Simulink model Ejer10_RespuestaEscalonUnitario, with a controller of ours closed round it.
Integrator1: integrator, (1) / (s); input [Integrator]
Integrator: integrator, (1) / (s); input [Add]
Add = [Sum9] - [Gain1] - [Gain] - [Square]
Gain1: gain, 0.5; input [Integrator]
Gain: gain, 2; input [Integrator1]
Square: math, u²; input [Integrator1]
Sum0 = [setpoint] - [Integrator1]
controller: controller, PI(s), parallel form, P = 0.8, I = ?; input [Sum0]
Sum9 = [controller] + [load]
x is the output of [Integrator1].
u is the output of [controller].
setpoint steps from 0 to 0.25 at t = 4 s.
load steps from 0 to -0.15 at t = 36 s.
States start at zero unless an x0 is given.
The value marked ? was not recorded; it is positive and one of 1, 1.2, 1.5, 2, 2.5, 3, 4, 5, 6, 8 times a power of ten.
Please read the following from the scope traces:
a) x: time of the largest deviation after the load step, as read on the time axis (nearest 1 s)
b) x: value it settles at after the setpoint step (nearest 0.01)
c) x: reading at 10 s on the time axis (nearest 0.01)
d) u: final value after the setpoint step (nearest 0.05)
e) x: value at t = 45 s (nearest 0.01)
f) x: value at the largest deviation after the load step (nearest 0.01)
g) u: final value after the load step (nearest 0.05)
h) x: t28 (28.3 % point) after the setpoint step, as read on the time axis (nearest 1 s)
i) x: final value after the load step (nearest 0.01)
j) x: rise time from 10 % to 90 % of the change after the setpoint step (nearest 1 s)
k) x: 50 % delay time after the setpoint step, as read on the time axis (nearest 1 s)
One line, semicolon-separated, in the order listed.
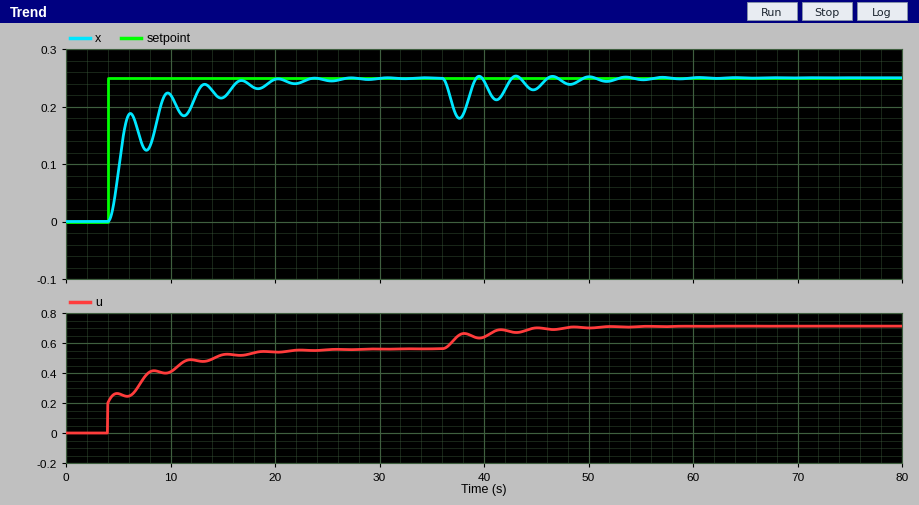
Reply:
38 s; 0.25; 0.22; 0.55; 0.23; 0.18; 0.70; 5 s; 0.25; 8 s; 5 s
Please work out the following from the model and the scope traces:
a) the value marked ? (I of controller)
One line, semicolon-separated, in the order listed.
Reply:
0.6
